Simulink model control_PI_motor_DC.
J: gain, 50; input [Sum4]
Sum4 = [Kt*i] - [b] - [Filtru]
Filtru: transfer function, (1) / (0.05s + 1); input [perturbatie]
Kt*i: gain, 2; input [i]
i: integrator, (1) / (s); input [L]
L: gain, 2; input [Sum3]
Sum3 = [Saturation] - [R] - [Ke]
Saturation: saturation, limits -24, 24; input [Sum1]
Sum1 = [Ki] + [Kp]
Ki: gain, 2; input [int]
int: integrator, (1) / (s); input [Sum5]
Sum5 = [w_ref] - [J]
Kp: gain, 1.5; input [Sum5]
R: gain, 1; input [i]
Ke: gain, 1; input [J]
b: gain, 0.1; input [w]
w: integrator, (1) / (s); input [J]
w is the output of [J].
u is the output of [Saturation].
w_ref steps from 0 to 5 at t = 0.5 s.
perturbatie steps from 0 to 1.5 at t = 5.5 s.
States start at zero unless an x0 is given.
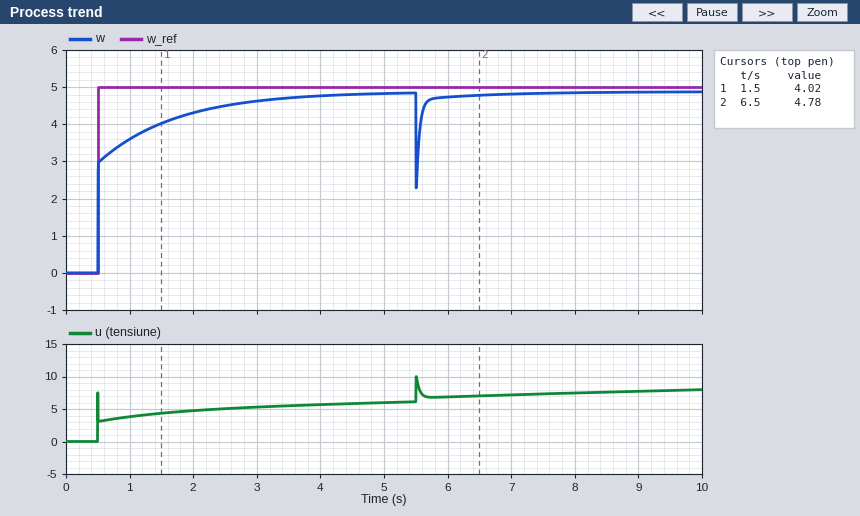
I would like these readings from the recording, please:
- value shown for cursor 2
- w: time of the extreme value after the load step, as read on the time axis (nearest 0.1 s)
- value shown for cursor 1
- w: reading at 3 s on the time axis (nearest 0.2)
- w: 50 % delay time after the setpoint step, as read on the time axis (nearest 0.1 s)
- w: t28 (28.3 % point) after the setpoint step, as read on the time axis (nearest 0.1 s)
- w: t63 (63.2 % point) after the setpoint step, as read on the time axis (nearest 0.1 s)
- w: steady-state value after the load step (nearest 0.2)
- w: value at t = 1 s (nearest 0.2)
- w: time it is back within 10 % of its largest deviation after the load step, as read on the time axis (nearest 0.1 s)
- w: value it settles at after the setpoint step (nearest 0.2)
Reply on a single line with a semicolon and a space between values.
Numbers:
4.78; 5.5 s; 4.02; 4.6; 0.5 s; 0.5 s; 0.6 s; 4.8; 3.6; 5.7 s; 4.8
